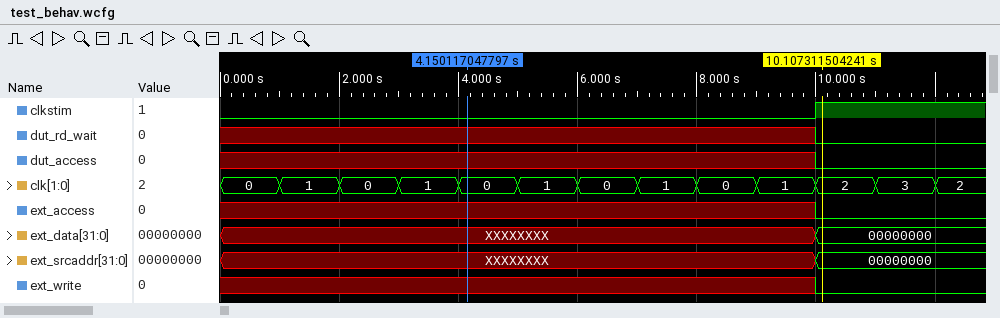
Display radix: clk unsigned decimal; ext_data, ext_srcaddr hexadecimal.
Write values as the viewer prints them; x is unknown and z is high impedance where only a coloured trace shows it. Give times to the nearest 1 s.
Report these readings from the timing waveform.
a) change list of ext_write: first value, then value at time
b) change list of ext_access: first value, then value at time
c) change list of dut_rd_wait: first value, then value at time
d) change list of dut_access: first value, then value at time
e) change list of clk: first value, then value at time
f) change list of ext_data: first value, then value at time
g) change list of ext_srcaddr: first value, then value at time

x, 0 at 10 s
x, 0 at 10 s
x, 0 at 10 s
x, 0 at 10 s
0, 1 at 1 s, 0 at 2 s, 1 at 3 s, 0 at 4 s, 1 at 5 s, 0 at 6 s, 1 at 7 s, 0 at 8 s, 1 at 9 s, 2 at 10 s, 3 at 11 s, 2 at 12 s
XXXXXXXX, 00000000 at 10 s
XXXXXXXX, 00000000 at 10 s
